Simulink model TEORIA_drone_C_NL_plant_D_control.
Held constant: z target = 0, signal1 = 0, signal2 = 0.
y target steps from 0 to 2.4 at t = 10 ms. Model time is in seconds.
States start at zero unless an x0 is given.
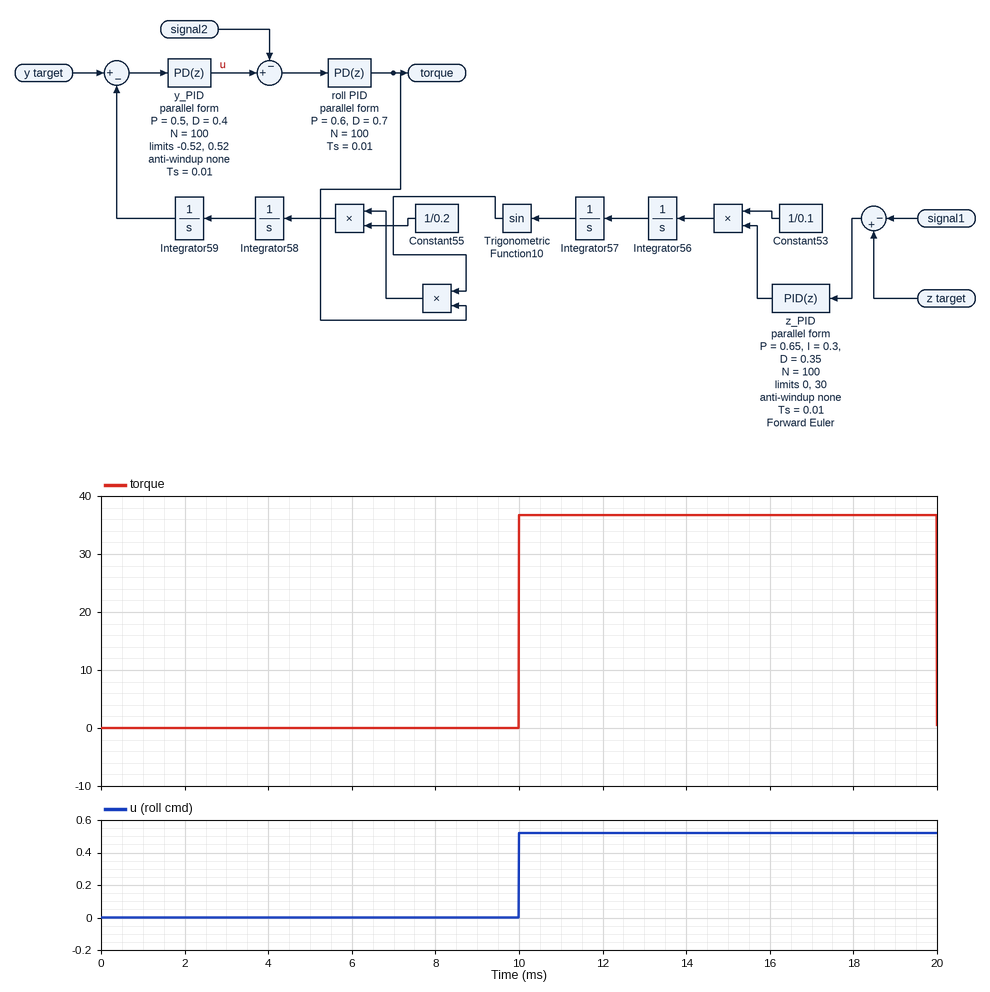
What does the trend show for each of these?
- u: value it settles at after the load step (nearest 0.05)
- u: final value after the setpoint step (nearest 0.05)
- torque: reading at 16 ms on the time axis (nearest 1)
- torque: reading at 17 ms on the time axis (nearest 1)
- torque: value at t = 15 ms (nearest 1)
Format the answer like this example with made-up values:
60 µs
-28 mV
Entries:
0.50
0.50
37
37
37
